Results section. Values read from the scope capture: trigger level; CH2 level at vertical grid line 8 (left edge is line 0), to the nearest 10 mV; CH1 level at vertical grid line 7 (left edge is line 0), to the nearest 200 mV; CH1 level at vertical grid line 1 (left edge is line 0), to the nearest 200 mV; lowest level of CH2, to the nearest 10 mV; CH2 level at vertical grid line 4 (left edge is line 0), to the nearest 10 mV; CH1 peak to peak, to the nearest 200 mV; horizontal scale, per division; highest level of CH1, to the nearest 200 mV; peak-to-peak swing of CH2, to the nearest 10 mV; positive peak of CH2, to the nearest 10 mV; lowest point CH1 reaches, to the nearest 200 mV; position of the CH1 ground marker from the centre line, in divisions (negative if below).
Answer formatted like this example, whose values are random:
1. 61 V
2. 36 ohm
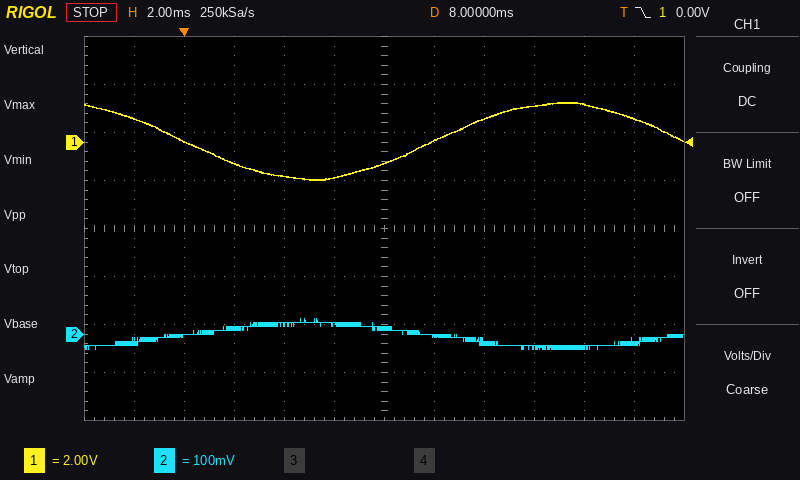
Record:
1. 0.00 V
2. -20 mV
3. 0.0 V
4. 1.0 V
5. -30 mV
6. 20 mV
7. 3.2 V
8. 2 ms
9. 1.6 V
10. 60 mV
11. 30 mV
12. -1.6 V
13. +1.8 div
